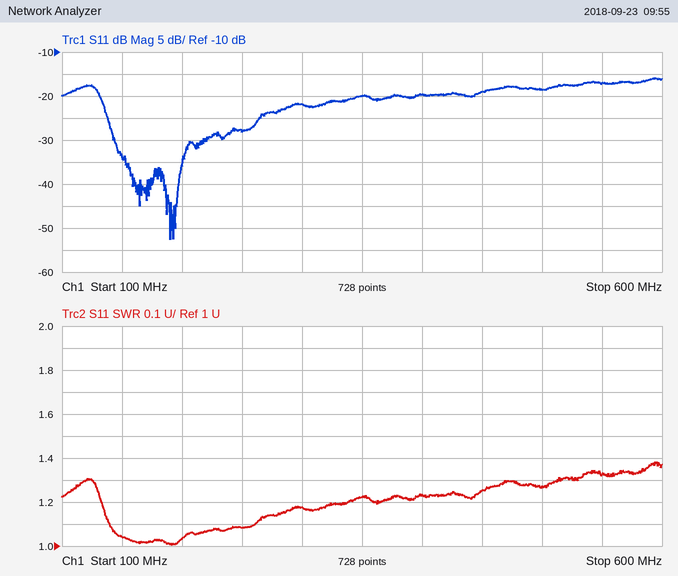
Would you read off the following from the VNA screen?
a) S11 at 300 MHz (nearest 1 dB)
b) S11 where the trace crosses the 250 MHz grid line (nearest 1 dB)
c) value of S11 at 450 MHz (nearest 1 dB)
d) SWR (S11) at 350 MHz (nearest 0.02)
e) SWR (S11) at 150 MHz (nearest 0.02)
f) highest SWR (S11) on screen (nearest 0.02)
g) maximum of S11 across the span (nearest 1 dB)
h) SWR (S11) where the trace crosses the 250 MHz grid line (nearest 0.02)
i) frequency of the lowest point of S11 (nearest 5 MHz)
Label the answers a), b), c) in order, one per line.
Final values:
a) -22 dB
b) -28 dB
c) -19 dB
d) 1.22
e) 1.04
f) 1.38
g) -16 dB
h) 1.08
i) 190 MHz
